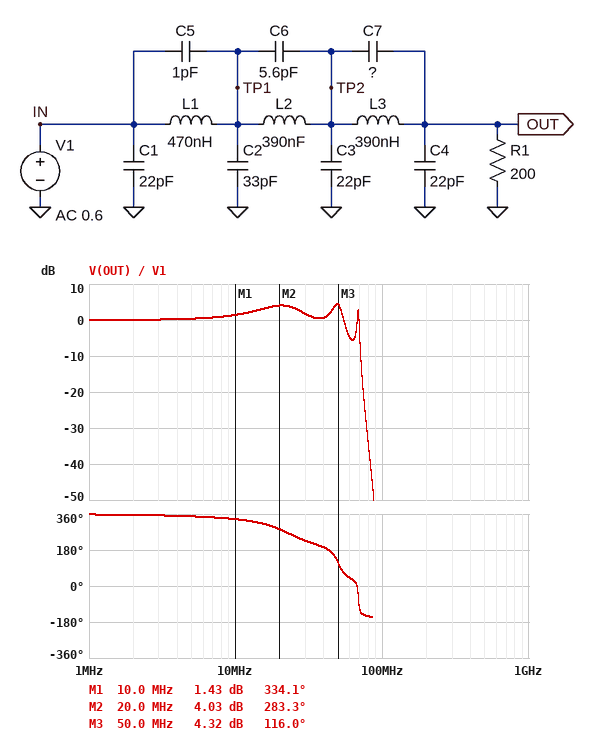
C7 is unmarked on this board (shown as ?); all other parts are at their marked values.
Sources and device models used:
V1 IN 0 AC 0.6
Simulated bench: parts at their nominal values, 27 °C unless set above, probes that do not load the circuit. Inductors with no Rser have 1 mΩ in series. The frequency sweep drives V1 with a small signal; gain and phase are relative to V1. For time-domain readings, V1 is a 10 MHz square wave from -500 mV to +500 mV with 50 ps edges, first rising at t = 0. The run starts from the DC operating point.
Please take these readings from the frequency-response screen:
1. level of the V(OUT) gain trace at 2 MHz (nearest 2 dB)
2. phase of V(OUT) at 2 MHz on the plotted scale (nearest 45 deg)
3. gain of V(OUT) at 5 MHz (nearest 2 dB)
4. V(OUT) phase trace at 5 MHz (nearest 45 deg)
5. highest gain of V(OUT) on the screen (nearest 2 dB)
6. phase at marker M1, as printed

0 dB
360 deg
0 dB
360 deg
4 dB
334.1 deg
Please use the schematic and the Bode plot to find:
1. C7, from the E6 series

6.8 pF
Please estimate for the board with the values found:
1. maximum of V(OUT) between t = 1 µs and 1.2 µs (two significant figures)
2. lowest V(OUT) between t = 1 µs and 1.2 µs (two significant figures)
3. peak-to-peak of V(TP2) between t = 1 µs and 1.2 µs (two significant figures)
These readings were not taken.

1.0 V
-1.0 V
1.8 V
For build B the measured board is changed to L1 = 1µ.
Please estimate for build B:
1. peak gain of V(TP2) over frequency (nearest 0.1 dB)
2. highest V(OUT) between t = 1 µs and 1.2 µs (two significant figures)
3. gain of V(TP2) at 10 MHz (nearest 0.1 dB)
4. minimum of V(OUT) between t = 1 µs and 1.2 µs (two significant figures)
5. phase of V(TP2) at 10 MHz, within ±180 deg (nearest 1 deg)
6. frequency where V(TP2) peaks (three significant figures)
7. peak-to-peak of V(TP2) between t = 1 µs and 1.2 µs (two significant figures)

2.5 dB
770 mV
1.7 dB
-770 mV
-33 deg
14.2 MHz
1.5 V
